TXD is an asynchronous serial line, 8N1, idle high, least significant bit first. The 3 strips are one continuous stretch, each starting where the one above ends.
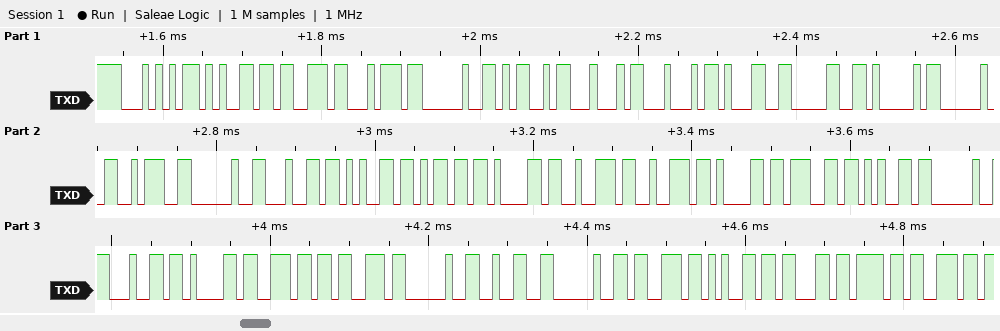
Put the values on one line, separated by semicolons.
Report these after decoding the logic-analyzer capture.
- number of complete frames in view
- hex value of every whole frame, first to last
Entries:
36; 54 65 73 74 20 4D 44 44 31 30 41 20 3A 20 64 65 6D 61 72 72 61 67 65 20 64 61 6E 73 20 32 20 73 65 63 6F 6E
